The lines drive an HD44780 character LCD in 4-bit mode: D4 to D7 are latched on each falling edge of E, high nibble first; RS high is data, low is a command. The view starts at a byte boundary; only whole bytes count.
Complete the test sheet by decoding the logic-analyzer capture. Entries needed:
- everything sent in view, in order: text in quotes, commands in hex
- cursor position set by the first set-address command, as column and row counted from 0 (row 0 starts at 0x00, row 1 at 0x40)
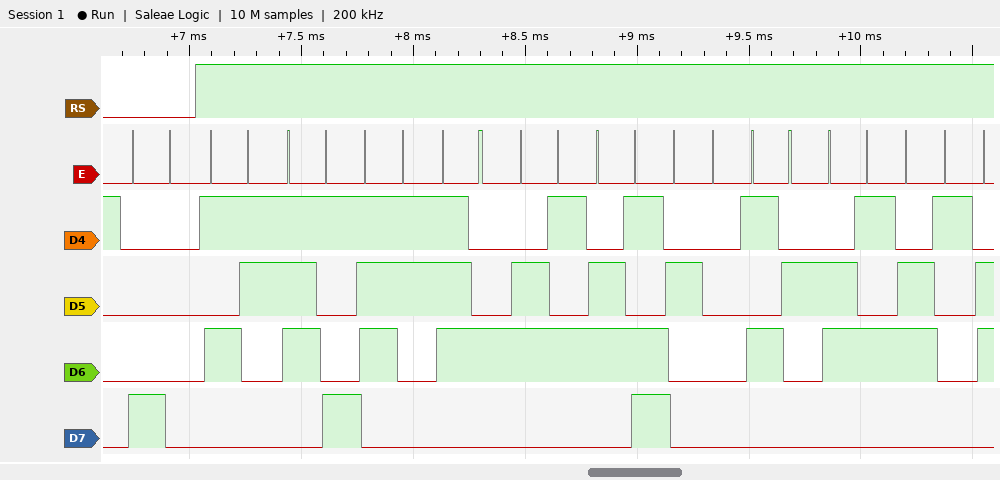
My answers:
0x80 "System Rea"
column 0, row 0
